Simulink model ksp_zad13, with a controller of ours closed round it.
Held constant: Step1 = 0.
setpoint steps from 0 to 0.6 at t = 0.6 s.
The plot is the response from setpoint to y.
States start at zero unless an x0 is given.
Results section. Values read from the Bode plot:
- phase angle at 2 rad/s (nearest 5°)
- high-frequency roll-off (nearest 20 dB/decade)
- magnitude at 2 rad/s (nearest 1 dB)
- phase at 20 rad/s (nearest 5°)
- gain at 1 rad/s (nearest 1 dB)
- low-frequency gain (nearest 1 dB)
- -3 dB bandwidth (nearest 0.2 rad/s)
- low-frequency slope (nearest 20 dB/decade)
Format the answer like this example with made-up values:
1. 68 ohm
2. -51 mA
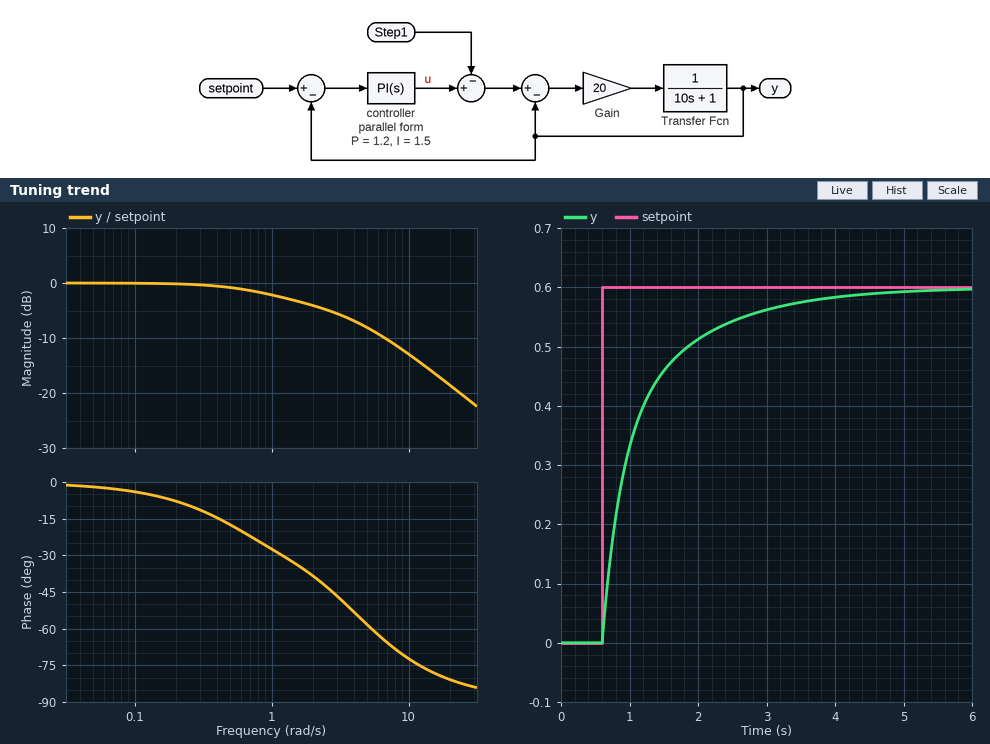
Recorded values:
1. -40°
2. -20 dB/decade
3. -4 dB
4. -80°
5. -2 dB
6. 0 dB
7. 1.4 rad/s
8. 0 dB/decade
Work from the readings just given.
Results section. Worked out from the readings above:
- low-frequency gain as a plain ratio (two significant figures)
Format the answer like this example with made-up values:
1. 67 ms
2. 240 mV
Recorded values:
1. 1.0
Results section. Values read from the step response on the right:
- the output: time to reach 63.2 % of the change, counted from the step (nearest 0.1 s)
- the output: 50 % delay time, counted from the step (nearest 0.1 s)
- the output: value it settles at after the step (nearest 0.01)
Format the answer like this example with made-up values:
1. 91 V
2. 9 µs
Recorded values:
1. 0.5 s
2. 0.3 s
3. 0.60
